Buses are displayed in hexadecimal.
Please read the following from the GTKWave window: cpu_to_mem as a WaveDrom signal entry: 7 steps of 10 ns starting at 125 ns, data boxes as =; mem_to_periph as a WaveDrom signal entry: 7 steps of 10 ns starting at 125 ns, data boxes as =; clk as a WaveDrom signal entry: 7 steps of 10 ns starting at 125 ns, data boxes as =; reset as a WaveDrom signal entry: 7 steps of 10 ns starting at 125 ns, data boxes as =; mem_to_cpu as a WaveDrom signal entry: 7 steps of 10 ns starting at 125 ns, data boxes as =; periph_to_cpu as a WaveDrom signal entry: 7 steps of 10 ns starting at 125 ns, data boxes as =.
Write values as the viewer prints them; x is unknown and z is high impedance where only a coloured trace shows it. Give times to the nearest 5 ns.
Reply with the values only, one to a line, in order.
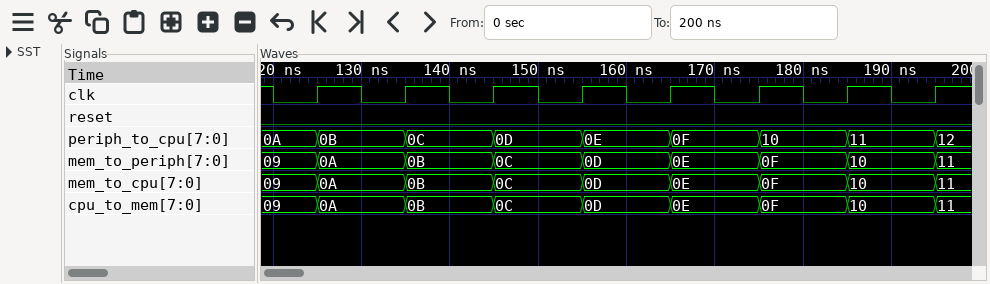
{name: 'cpu_to_mem', wave: '=======', data: '0A 0B 0C 0D 0E 0F 10'}
{name: 'mem_to_periph', wave: '=======', data: '0A 0B 0C 0D 0E 0F 10'}
{name: 'clk', wave: 'p......'}
{name: 'reset', wave: '0......'}
{name: 'mem_to_cpu', wave: '=======', data: '0A 0B 0C 0D 0E 0F 10'}
{name: 'periph_to_cpu', wave: '=======', data: '0B 0C 0D 0E 0F 10 11'}
